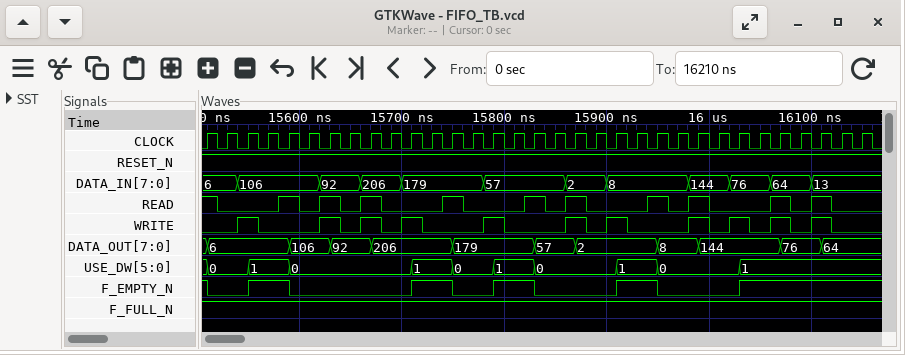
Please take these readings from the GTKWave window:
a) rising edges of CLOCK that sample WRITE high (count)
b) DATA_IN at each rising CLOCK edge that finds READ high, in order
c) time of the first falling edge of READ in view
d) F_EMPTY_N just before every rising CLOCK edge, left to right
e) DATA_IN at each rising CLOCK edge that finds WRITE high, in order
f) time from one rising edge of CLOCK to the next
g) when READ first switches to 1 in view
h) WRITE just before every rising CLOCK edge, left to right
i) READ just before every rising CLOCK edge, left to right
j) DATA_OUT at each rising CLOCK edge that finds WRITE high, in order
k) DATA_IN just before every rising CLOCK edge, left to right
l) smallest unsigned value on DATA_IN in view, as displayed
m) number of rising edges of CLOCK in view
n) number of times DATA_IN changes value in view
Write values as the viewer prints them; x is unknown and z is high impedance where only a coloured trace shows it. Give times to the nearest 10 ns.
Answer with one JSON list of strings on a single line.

["11", "6, 106, 92, 206, 179, 57, 2, 8, 144, 64, 13", "15520 ns", "1 0 0 1 1 0 0 0 0 0 0 1 1 0 0 1 1 0 0 0 0 1 1 0 0 0 0 1 1 1 1 1 1", "106, 92, 206, 179, 57, 2, 8, 144, 76, 64, 13", "20 ns", "15580 ns", "0 0 1 0 0 0 1 0 1 0 1 0 0 0 1 0 0 0 1 0 1 0 0 0 1 0 1 0 1 0 1 0 0", "1 0 0 0 1 0 1 0 1 0 0 0 1 0 0 0 1 0 1 0 0 0 1 0 1 0 0 0 1 0 1 0 0", "6, 106, 92, 206, 179, 57, 2, 8, 144, 144, 76", "6, 6, 106, 106, 106, 106, 92, 92, 206, 206, 179, 179, 179, 179, 57, 57, 57, 57, 2, 2, 8, 8, 8, 8, 144, 144, 76, 76, 64, 64, 13, 13, 13", "2", "33", "11"]
